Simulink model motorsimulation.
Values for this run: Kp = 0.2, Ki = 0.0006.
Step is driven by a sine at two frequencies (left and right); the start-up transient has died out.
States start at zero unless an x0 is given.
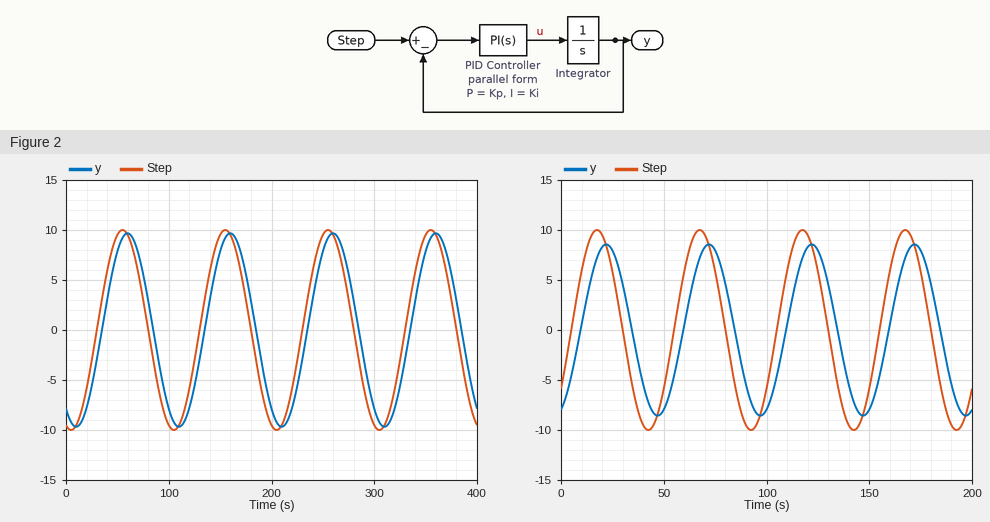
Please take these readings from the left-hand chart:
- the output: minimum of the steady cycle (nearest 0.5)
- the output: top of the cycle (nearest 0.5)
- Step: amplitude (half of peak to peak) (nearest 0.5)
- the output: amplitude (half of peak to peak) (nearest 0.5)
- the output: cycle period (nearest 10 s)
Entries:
-9.5
9.5
10.0
9.5
100 s
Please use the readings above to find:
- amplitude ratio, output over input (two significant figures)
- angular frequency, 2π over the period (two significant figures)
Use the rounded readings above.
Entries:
0.95
0.063 rad/s
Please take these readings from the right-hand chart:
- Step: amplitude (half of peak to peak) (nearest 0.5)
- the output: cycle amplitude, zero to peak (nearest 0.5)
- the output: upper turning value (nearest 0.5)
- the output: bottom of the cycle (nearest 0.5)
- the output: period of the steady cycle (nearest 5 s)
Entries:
10.0
8.5
8.5
-8.5
50 s
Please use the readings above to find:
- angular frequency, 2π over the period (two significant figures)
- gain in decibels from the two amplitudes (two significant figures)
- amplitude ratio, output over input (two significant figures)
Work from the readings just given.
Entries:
0.13 rad/s
-1.4 dB
0.85
